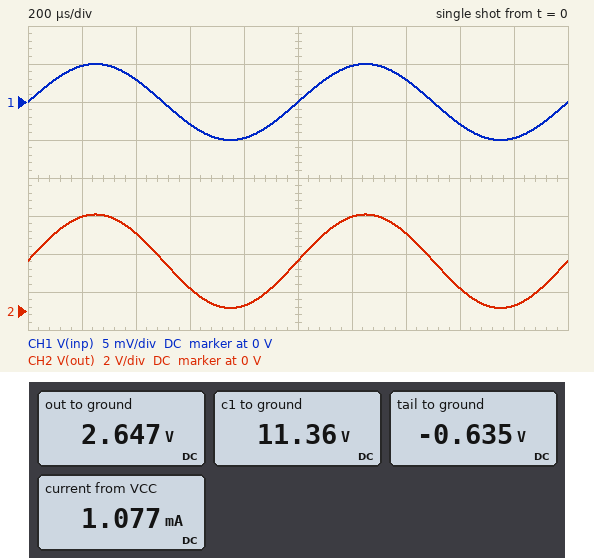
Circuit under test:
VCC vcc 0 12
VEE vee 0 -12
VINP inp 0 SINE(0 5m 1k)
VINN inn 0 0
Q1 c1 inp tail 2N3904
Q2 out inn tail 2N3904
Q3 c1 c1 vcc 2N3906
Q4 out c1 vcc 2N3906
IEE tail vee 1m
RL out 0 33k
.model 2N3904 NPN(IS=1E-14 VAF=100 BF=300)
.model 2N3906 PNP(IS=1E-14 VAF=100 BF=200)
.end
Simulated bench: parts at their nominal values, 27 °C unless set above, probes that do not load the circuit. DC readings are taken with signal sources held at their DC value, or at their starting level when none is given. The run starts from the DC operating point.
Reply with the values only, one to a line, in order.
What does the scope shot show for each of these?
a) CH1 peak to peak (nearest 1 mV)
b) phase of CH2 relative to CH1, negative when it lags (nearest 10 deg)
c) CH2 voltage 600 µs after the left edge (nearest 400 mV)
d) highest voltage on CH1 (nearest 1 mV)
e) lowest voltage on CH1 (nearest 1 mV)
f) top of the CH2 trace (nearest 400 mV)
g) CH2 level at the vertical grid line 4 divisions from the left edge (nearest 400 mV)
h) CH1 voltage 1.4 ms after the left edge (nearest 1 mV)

10 mV
0 deg
1.2 V
5 mV
-5 mV
5.2 V
400 mV
3 mV
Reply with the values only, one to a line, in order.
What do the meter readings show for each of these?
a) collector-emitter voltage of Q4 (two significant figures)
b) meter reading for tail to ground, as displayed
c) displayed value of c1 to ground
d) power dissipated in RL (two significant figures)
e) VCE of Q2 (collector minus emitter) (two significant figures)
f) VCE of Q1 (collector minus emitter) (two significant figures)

-9.4 V
-0.635 V
11.36 V
210 µW
3.3 V
12 V
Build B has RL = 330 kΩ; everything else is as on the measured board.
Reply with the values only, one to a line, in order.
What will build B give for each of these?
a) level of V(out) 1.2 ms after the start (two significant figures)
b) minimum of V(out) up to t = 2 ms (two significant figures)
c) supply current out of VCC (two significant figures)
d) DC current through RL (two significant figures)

12 V
490 mV
1.0 mA
25 µA
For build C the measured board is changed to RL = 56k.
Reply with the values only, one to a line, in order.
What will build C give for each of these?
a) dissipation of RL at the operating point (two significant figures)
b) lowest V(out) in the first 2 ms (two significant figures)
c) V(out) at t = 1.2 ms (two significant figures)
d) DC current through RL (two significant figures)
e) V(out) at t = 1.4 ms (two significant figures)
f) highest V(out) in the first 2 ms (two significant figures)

260 µW
230 mV
7.2 V
68 µA
5.9 V
7.3 V
